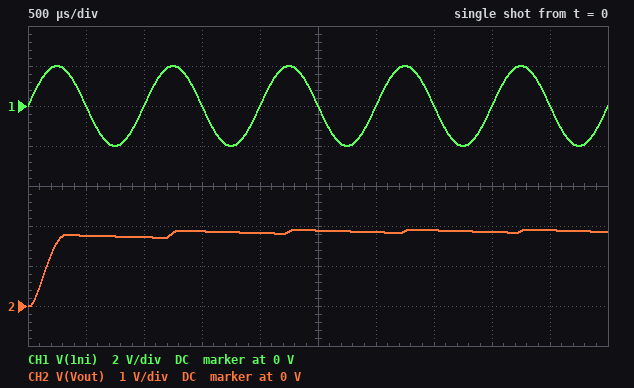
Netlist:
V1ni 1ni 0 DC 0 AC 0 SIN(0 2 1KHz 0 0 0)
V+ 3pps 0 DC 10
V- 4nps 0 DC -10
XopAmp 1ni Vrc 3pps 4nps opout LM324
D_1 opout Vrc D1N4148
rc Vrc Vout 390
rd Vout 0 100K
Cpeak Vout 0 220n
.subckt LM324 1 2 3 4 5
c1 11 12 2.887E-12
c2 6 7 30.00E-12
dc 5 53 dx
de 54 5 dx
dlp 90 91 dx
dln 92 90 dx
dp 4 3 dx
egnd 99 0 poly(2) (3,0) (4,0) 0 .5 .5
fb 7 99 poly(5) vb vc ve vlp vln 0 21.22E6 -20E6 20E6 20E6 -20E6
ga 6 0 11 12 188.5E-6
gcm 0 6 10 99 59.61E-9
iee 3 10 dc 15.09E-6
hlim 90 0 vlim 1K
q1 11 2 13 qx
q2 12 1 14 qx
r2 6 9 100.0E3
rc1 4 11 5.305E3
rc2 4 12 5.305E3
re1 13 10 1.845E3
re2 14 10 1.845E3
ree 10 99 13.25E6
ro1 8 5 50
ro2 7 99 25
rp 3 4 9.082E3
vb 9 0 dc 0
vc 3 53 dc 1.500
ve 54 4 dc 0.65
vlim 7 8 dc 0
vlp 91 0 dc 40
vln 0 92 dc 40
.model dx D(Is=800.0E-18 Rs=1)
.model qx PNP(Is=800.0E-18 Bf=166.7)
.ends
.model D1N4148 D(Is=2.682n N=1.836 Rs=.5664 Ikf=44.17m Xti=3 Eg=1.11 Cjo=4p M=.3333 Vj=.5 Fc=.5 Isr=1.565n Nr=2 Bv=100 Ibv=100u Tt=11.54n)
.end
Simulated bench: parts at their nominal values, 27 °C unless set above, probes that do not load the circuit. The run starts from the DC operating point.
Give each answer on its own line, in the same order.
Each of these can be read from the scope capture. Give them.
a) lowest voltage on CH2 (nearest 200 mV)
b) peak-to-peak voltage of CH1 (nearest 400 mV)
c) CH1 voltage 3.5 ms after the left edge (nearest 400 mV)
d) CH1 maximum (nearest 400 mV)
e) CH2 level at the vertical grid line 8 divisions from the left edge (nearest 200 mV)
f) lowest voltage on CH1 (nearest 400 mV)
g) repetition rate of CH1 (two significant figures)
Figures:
0 V
4.0 V
0 V
2.0 V
1.8 V
-2.0 V
1.0 kHz
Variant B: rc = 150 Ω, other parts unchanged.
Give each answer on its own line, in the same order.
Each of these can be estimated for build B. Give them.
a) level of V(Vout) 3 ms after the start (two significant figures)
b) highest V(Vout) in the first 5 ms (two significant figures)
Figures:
1.9 V
2.0 V
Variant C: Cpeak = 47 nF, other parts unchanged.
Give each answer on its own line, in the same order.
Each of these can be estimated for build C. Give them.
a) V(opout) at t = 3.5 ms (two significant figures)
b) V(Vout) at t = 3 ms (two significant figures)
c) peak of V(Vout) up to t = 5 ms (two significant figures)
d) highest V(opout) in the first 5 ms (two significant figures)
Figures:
-10 V
1.7 V
2.0 V
2.5 V
